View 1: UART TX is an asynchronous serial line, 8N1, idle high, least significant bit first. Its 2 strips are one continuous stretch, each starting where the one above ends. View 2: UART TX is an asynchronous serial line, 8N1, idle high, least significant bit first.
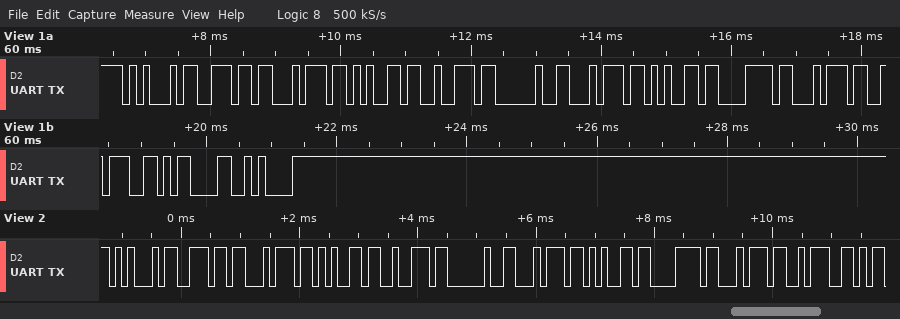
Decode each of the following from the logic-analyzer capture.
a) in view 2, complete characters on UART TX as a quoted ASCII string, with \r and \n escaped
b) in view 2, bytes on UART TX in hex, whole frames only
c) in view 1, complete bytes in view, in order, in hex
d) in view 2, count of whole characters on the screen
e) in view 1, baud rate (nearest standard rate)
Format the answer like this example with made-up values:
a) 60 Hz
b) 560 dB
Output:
a) "Enter text:"
b) 0x45 0x6E 0x74 0x65 0x72 0x20 0x74 0x65 0x78 0x74 0x3A
c) 45 6E 74 65 72 20 74 65 78 74 3A 0D 0A
d) 11
e) 9600 baud
